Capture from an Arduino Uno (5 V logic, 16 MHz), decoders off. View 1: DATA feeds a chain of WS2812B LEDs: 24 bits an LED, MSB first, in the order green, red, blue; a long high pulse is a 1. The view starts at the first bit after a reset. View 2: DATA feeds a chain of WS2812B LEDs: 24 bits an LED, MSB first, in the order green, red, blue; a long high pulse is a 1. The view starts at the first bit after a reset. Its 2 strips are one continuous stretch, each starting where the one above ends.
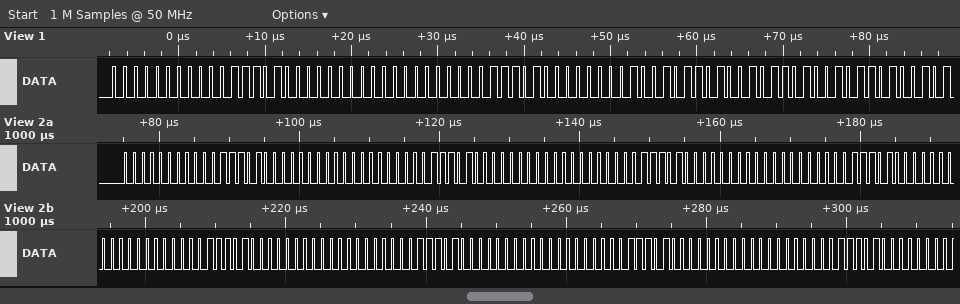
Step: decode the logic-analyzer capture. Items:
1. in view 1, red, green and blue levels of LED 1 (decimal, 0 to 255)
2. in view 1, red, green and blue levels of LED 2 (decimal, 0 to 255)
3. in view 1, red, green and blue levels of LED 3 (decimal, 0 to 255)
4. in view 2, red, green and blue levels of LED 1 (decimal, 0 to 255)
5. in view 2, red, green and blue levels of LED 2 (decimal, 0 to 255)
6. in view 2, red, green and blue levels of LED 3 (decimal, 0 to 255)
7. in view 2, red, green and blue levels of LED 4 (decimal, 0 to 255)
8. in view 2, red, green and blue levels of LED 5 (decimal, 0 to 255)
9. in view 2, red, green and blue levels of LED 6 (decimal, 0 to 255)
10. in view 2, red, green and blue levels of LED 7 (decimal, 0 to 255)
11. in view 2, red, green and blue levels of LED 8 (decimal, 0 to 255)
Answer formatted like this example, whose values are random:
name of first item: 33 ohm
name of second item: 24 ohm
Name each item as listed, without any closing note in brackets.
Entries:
in view 1, red, green and blue levels of LED 1: 29, 0, 0
in view 1, red, green and blue levels of LED 2: 29, 0, 0
in view 1, red, green and blue levels of LED 3: 150, 150, 150
in view 2, red, green and blue levels of LED 1: 29, 0, 0
in view 2, red, green and blue levels of LED 2: 29, 0, 0
in view 2, red, green and blue levels of LED 3: 29, 0, 0
in view 2, red, green and blue levels of LED 4: 29, 0, 0
in view 2, red, green and blue levels of LED 5: 29, 0, 0
in view 2, red, green and blue levels of LED 6: 29, 0, 0
in view 2, red, green and blue levels of LED 7: 29, 0, 0
in view 2, red, green and blue levels of LED 8: 29, 0, 0
